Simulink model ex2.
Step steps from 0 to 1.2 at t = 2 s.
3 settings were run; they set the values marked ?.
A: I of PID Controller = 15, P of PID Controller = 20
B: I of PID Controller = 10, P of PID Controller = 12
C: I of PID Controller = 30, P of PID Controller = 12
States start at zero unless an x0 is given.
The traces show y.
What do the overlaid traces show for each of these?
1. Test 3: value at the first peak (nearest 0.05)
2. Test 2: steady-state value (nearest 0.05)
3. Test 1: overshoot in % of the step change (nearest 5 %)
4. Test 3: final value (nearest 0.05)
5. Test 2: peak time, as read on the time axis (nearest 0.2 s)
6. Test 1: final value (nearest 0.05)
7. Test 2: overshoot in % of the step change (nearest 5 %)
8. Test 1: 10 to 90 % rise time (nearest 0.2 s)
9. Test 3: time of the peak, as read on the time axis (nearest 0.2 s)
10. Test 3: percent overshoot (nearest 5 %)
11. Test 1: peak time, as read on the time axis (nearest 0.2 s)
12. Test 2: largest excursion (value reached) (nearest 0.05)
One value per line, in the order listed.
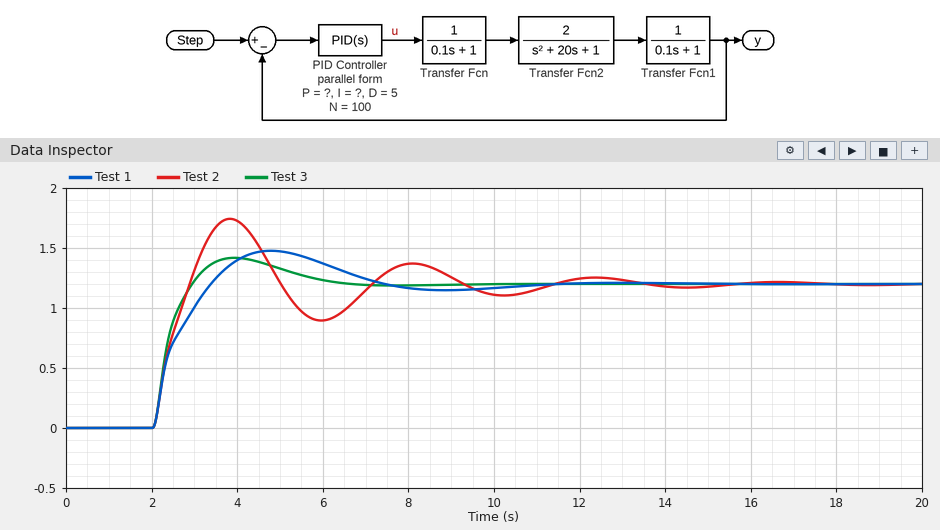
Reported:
1.40
1.20
25 %
1.20
3.8 s
1.20
45 %
1.0 s
4.0 s
20 %
4.8 s
1.75
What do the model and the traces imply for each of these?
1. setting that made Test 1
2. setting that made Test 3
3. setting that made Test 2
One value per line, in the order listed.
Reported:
B
A
C
